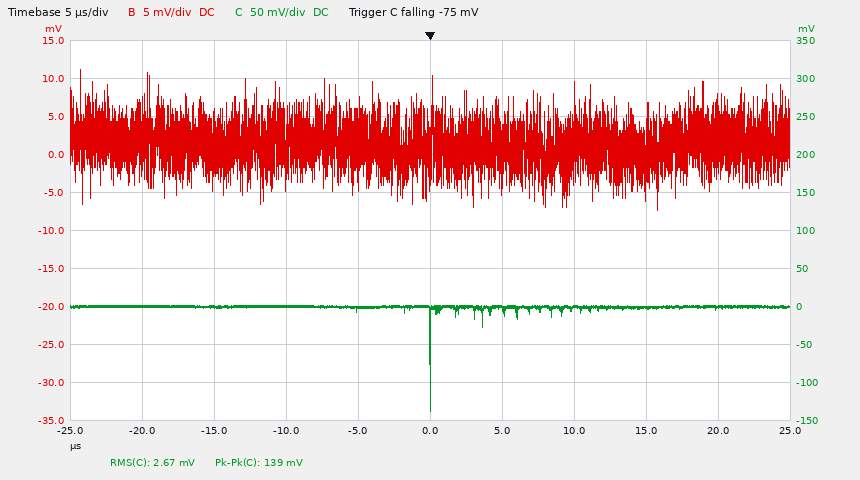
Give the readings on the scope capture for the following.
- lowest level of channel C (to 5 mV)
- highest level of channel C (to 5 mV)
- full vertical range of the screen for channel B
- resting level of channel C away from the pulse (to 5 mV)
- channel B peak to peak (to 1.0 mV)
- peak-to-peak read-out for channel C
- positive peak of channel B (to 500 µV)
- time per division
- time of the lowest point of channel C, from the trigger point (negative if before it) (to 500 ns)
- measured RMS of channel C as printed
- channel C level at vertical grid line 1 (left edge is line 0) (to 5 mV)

-135 mV
0 mV
50 mV
0 mV
18.0 mV
139 mV
11.0 mV
5 µs
0.0 µs
2.67 mV
0 mV
